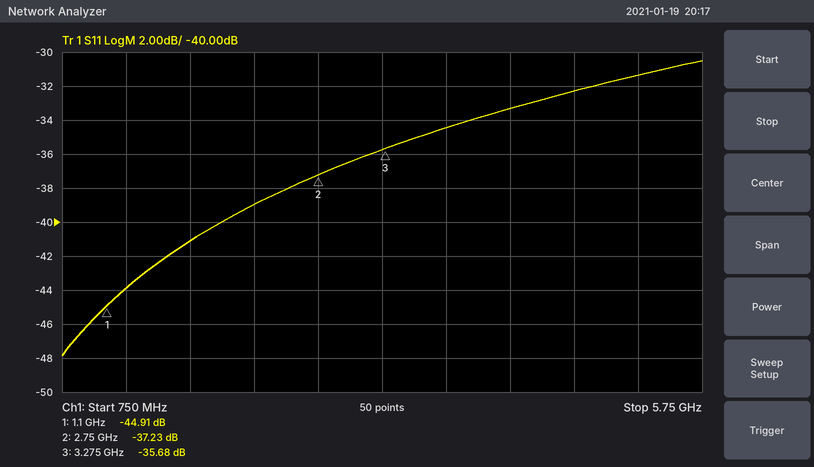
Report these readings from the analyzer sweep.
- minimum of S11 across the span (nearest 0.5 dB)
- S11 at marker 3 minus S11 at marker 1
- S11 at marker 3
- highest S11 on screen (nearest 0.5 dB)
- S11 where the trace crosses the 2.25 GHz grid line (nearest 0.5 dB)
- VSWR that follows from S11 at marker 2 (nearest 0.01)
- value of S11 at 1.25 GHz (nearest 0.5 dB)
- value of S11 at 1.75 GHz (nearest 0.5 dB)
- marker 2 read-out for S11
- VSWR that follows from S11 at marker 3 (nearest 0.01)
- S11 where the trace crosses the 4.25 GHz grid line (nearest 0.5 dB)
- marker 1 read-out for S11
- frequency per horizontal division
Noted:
-48.0 dB
9.23 dB
-35.68 dB
-30.5 dB
-39.0 dB
1.03
-44.0 dB
-41.0 dB
-37.23 dB
1.03
-33.5 dB
-44.91 dB
500 MHz
